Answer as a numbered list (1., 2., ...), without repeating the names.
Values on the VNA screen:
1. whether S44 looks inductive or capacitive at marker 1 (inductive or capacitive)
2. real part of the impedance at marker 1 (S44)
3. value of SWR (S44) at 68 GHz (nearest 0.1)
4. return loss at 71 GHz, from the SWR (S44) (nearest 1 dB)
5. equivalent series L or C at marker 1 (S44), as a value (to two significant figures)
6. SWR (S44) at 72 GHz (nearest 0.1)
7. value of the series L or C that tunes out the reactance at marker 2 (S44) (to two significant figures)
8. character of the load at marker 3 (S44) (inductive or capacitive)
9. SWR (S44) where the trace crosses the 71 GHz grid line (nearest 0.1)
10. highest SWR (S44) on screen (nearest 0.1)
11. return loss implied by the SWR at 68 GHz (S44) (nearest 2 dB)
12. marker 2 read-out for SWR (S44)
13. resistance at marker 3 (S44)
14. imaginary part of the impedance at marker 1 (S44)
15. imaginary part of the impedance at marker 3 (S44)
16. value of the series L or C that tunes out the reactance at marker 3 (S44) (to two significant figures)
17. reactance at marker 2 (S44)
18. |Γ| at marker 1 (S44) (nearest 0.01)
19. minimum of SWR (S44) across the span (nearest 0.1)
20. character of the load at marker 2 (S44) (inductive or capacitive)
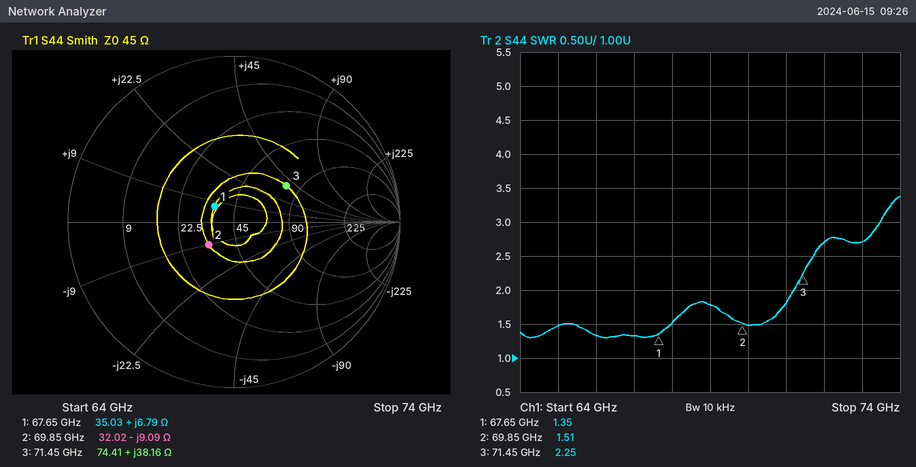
1. inductive
2. 35.03 Ω
3. 1.5
4. 11 dB
5. 16 pH
6. 2.7
7. 21 pH
8. inductive
9. 1.8
10. 3.4
11. 14 dB
12. 1.51
13. 74.41 Ω
14. +6.79 Ω
15. +38.16 Ω
16. 58 fF
17. -9.09 Ω
18. 0.15
19. 1.3
20. capacitive
